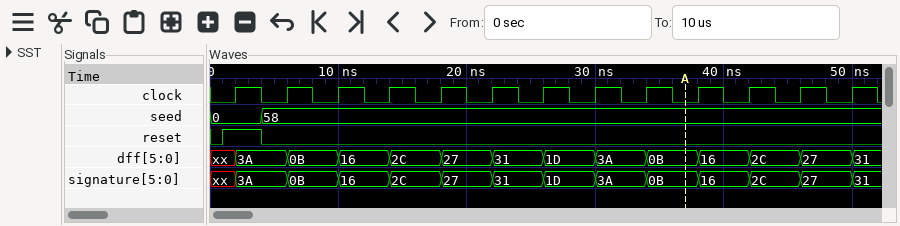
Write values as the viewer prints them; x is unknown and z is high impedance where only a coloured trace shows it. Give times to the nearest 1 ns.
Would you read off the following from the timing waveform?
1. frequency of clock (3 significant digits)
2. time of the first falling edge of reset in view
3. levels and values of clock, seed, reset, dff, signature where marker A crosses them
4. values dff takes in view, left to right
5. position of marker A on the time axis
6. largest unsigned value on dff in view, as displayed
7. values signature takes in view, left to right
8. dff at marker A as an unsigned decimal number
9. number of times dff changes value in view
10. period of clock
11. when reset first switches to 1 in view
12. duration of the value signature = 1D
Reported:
250 MHz
4 ns
clock=0, seed=58, reset=0, dff=0B, signature=0B
xx, 3A, 0B, 16, 2C, 27, 31, 1D, 3A, 0B, 16, 2C, 27, 31
37 ns
3A
xx, 3A, 0B, 16, 2C, 27, 31, 1D, 3A, 0B, 16, 2C, 27, 31
11
13
4 ns
1 ns
4 ns
